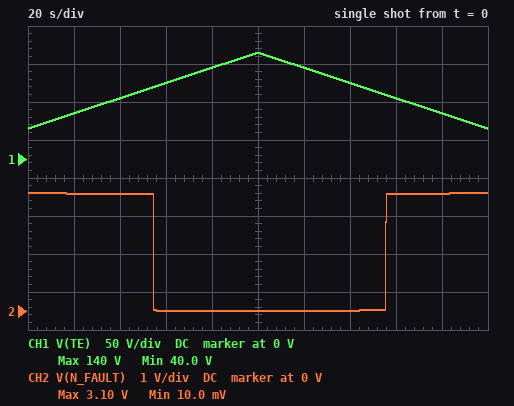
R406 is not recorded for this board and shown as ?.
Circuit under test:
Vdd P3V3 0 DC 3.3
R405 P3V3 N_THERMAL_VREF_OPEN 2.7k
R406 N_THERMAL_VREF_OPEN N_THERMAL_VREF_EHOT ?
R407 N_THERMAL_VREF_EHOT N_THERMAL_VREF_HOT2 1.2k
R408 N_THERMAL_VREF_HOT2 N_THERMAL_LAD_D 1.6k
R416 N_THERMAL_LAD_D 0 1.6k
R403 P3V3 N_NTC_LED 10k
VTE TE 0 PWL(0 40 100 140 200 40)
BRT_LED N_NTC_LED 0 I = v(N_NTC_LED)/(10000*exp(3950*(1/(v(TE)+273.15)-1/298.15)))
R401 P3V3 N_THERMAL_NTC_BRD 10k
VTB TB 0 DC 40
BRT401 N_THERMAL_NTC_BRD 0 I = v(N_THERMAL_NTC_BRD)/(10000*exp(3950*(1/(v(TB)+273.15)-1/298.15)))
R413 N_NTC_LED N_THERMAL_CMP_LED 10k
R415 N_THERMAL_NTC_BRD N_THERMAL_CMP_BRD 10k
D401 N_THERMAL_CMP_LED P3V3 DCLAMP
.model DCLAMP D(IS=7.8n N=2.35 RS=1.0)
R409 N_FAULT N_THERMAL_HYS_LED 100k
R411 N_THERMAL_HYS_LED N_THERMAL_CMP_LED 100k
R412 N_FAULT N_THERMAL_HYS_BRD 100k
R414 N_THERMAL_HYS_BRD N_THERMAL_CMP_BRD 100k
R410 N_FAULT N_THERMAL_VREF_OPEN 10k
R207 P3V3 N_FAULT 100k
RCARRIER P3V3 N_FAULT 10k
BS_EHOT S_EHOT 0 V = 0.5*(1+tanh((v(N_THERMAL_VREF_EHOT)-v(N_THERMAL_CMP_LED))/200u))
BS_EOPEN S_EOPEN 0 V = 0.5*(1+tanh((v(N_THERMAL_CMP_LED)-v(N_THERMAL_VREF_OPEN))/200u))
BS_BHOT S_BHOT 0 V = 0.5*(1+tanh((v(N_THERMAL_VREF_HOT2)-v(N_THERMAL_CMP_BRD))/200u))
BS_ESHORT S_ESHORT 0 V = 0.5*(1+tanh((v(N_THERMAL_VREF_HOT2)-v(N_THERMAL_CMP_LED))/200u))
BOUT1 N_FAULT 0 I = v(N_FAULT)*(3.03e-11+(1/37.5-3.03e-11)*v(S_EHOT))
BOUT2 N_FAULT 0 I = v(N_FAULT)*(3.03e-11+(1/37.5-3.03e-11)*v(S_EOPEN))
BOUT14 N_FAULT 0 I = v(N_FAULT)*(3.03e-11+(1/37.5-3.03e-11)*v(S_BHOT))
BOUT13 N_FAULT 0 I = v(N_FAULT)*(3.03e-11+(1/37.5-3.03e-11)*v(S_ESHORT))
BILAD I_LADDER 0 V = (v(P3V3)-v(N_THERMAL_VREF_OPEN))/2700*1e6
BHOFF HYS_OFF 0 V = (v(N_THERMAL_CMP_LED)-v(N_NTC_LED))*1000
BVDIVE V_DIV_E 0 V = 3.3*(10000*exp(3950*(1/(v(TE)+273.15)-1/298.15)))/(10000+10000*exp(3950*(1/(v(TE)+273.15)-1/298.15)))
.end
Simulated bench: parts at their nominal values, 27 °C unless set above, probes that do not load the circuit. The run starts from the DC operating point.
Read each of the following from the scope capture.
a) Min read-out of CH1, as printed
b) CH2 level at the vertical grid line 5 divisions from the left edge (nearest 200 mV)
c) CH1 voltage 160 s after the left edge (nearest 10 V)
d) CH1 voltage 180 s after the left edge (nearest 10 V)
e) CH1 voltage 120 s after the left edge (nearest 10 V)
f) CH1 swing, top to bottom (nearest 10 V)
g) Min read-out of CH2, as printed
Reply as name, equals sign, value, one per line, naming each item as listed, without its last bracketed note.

Min read-out of CH1, as printed = 40.0 V
CH2 level at the vertical grid line 5 divisions from the left edge = 0 V
CH1 voltage 160 s after the left edge = 80 V
CH1 voltage 180 s after the left edge = 60 V
CH1 voltage 120 s after the left edge = 120 V
CH1 swing, top to bottom = 100 V
Min read-out of CH2, as printed = 10.0 mV
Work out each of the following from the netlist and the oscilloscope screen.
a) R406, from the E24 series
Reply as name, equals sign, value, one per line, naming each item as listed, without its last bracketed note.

R406, from the E24 series = 30 kΩ
